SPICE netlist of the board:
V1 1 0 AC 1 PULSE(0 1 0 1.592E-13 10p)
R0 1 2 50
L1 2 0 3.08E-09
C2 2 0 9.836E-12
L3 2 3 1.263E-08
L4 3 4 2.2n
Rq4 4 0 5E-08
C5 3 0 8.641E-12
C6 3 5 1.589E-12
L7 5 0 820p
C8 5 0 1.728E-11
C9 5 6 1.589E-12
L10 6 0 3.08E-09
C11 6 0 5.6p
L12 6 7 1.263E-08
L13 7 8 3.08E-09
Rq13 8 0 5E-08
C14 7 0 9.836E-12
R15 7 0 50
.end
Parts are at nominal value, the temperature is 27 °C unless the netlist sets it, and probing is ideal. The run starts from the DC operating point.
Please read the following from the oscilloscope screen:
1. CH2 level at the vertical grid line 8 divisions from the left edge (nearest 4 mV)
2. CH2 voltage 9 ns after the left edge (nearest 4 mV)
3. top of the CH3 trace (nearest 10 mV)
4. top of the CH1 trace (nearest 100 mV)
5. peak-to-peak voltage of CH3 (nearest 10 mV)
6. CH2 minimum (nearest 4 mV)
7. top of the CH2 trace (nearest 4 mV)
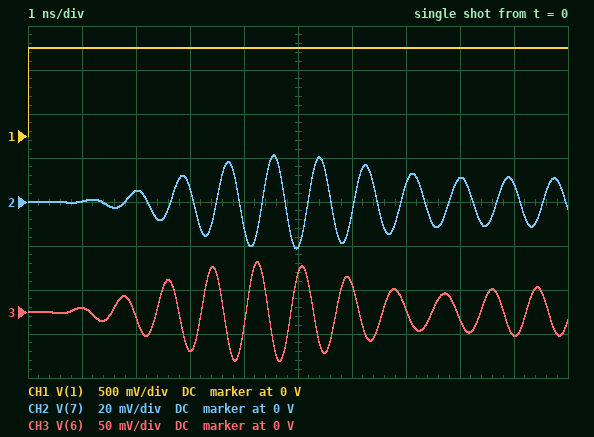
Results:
12 mV
8 mV
60 mV
1.0 V
110 mV
-20 mV
20 mV
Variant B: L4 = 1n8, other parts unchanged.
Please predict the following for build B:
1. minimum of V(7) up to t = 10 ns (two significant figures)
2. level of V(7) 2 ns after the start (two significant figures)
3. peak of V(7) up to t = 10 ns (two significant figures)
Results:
-19 mV
4.7 mV
19 mV
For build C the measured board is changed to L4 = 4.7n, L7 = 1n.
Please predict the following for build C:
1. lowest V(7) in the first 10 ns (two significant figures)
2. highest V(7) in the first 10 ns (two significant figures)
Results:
-11 mV
11 mV
